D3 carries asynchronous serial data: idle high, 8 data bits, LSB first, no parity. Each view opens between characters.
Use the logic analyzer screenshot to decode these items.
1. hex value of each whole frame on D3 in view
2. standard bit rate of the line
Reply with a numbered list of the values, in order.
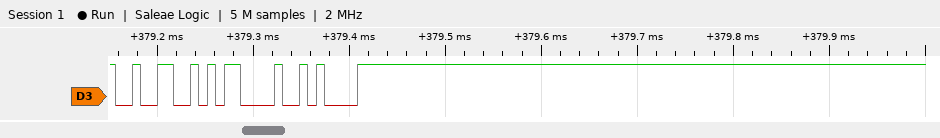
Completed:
1. 32, 0D, 0A
2. 115200 baud
